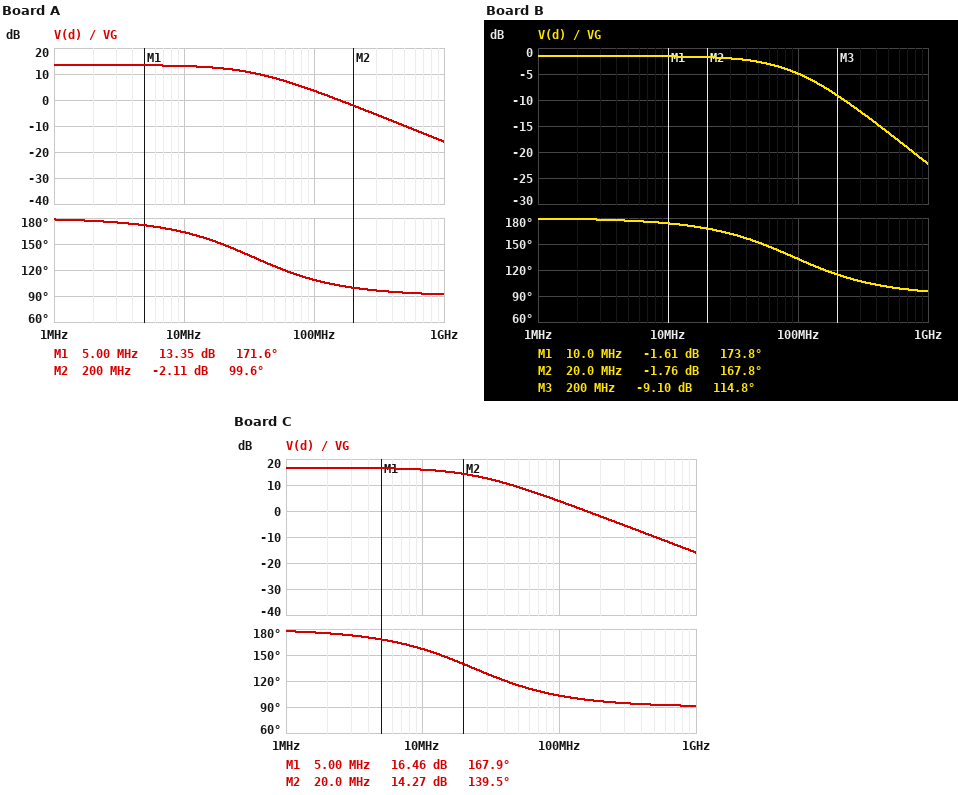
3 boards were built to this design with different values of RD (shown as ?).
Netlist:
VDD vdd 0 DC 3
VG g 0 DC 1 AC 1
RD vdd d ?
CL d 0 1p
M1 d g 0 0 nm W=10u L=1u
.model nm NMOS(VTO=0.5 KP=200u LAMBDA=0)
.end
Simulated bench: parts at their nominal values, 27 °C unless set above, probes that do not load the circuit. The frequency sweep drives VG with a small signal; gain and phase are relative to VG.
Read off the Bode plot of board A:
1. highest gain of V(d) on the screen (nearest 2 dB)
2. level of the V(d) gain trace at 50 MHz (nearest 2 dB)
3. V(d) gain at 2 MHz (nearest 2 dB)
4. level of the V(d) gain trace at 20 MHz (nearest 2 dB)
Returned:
14 dB
8 dB
14 dB
12 dB
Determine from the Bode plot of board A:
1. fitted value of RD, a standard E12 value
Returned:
4.7 kΩ
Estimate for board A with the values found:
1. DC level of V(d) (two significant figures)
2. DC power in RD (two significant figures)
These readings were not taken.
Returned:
1.8 V
290 µW
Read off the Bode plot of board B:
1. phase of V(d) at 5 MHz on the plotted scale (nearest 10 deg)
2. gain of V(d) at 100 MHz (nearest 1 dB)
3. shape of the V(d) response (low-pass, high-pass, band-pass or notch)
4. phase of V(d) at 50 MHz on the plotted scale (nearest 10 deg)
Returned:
180 deg
-5 dB
low-pass
150 deg
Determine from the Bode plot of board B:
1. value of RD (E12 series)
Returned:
15 kΩ
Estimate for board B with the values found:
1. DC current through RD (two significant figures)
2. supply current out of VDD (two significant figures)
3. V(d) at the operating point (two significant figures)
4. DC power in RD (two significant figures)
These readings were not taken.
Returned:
180 µA
180 µA
240 mV
510 µW
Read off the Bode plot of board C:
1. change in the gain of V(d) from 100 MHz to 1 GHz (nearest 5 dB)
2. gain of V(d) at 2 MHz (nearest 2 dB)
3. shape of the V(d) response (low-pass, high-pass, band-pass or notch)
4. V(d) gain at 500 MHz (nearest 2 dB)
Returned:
-20 dB
16 dB
low-pass
-10 dB
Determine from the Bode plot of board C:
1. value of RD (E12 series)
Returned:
6.8 kΩ
